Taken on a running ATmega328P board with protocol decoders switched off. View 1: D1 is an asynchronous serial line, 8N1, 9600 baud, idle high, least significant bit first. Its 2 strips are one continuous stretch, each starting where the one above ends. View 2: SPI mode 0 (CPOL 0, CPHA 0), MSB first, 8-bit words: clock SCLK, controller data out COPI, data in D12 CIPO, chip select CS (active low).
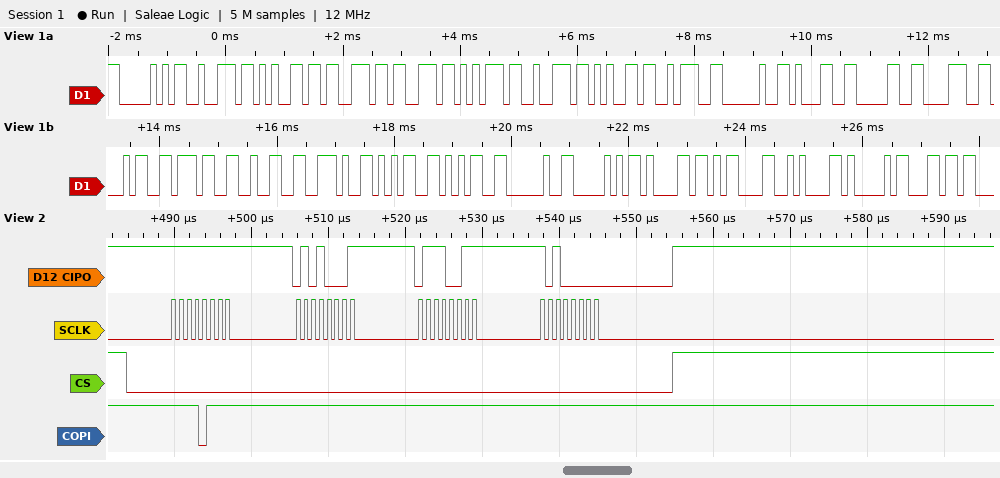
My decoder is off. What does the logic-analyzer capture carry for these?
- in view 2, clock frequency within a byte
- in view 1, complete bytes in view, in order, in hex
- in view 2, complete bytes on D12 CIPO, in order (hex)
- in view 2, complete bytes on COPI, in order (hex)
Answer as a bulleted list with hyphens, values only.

- 1 MHz
- 50 72 65 73 73 75 72 65 3A 20 31 30 38 34 37 32 2E 35 35 20 50 61 0D 0A 41 6C
- FF 51 73 A0
- F7 FF FF FF
